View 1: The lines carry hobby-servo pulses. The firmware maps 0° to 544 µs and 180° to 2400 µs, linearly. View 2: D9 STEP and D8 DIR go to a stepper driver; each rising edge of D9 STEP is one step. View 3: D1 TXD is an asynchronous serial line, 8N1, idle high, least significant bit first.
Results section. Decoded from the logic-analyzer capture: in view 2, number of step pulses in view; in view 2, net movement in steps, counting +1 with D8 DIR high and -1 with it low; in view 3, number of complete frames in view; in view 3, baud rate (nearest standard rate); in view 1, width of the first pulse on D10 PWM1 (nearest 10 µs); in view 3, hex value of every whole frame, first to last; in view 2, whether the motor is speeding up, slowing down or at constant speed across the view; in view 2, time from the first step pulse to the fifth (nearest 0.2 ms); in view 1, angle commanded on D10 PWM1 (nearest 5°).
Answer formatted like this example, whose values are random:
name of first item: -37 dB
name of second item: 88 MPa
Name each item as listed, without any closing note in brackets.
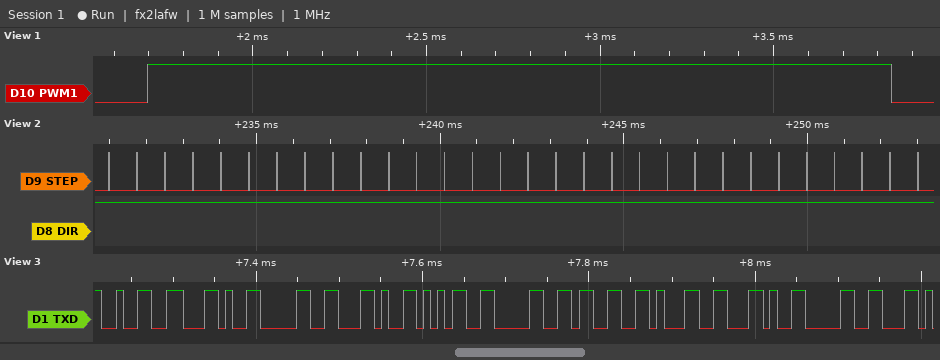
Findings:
in view 2, number of step pulses in view: 30
in view 2, net movement in steps, counting +1 with D8 DIR high and -1 with it low: +30
in view 3, number of complete frames in view: 10
in view 3, baud rate: 115200 baud
in view 1, width of the first pulse on D10 PWM1: 2140 µs
in view 3, hex value of every whole frame, first to last: 32 2C 30 2C 35 30 33 31 2C 30
in view 2, whether the motor is speeding up, slowing down or at constant speed across the view: constant speed
in view 2, time from the first step pulse to the fifth: 3.0 ms
in view 1, angle commanded on D10 PWM1: 155°
